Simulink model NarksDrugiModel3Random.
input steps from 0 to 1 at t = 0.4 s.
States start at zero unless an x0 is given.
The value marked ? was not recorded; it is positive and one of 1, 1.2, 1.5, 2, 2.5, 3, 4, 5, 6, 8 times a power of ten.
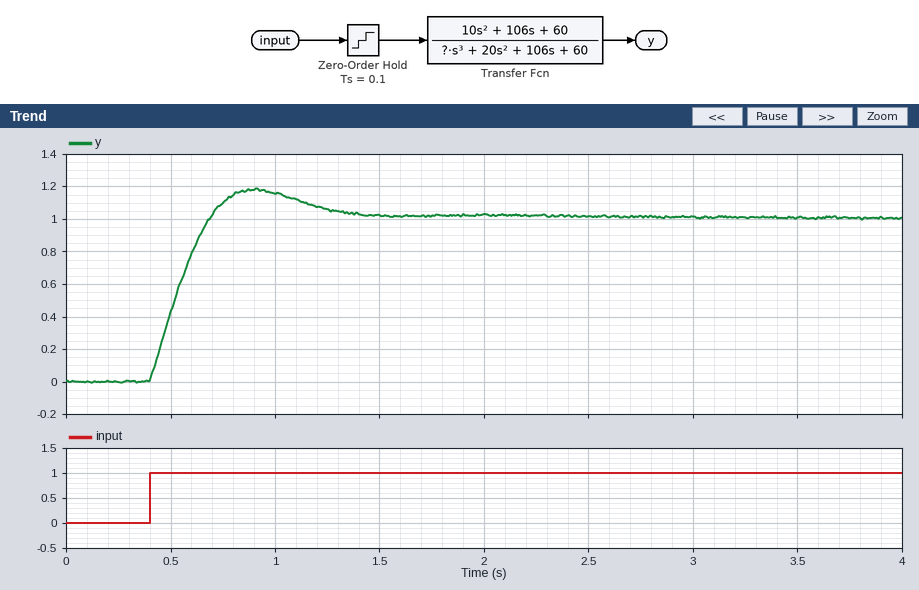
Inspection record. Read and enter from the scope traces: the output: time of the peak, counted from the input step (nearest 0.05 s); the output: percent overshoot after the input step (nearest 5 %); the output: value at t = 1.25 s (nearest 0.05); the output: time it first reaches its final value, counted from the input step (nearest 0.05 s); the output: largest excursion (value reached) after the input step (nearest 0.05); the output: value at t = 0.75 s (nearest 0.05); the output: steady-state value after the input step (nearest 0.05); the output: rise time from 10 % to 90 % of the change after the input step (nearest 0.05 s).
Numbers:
0.50 s
20 %
1.05
0.30 s
1.20
1.10
1.00
0.20 s
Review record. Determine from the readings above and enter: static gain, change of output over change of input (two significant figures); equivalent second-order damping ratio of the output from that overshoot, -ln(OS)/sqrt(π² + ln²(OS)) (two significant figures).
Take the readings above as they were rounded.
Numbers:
1.0
0.46
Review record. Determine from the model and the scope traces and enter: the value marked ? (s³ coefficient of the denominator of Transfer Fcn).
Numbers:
2.5
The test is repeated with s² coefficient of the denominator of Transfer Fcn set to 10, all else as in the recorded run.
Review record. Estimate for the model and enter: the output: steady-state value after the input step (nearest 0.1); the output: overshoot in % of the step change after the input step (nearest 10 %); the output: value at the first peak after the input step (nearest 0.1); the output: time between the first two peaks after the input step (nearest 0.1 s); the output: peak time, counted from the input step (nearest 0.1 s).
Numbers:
1.0
50 %
1.5
1.0 s
0.4 s
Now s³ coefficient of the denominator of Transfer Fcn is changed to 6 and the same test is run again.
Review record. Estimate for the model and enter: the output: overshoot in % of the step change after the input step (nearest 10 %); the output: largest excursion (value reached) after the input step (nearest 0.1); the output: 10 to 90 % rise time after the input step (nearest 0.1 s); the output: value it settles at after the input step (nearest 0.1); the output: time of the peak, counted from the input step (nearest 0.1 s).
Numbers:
40 %
1.4
0.3 s
1.0
0.7 s
